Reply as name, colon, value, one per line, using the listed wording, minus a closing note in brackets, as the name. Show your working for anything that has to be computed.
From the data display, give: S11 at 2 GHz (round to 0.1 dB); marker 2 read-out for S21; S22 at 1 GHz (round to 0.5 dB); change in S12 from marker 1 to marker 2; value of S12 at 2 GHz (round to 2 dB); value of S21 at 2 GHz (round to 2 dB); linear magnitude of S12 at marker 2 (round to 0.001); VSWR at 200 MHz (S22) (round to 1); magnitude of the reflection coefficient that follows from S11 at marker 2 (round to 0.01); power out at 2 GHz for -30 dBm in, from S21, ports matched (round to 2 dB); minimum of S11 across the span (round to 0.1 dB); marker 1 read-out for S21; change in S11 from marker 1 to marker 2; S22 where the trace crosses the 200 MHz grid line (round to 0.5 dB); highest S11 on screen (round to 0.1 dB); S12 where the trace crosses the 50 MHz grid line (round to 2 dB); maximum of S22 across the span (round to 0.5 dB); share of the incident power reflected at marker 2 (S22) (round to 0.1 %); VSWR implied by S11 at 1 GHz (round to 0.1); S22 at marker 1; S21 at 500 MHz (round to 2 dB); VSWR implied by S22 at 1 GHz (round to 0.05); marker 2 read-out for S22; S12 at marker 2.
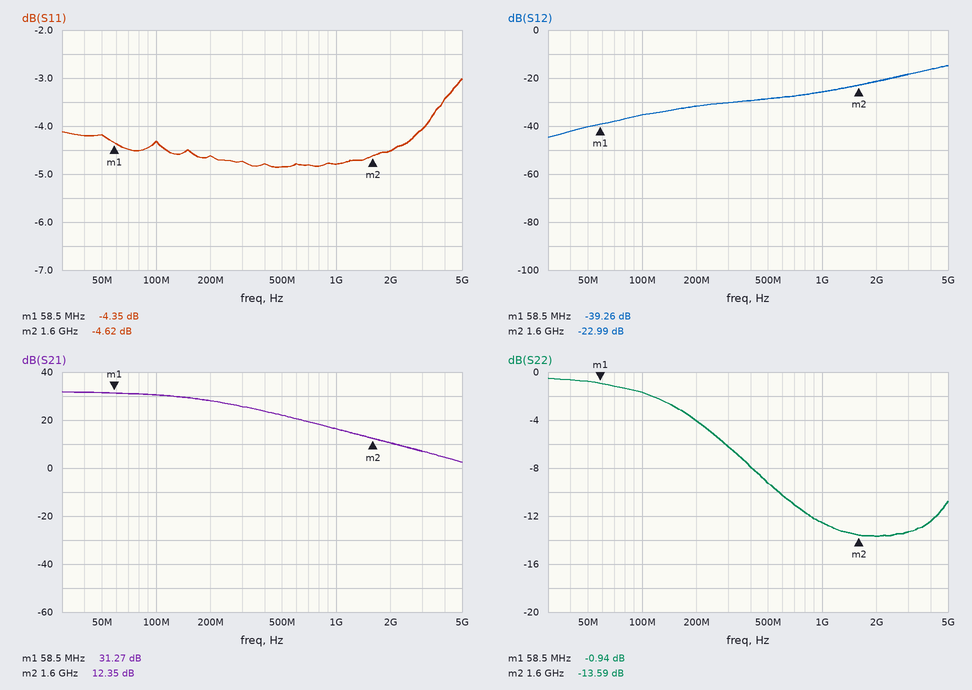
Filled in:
S11 at 2 GHz: -4.5 dB
marker 2 read-out for S21: 12.35 dB
S22 at 1 GHz: -12.5 dB
change in S12 from marker 1 to marker 2: -22.99 − (-39.26) = 16.27 dB
value of S12 at 2 GHz: -22 dB
value of S21 at 2 GHz: 10 dB
linear magnitude of S12 at marker 2: 10^(-22.99/20) ≈ 0.071
VSWR at 200 MHz (S22): |Γ| = 10^(-4/20) = 0.6310; VSWR = (1 + 0.6310)/(1 − 0.6310) ≈ 4
magnitude of the reflection coefficient that follows from S11 at marker 2: 10^(-4.62/20) ≈ 0.59
power out at 2 GHz for -30 dBm in, from S21, ports matched: -30 dBm + (10 dB) = -20 dBm
minimum of S11 across the span: -4.9 dB
marker 1 read-out for S21: 31.27 dB
change in S11 from marker 1 to marker 2: -4.62 − (-4.35) = -0.27 dB
S22 where the trace crosses the 200 MHz grid line: -4.0 dB
highest S11 on screen: -3.0 dB
S12 where the trace crosses the 50 MHz grid line: -40 dB
maximum of S22 across the span: -0.5 dB
share of the incident power reflected at marker 2 (S22): 10^(-13.59/10) ≈ 4.4 %
VSWR implied by S11 at 1 GHz: |Γ| = 10^(-4.8/20) = 0.5754; VSWR = (1 + 0.5754)/(1 − 0.5754) ≈ 3.7
S22 at marker 1: -0.94 dB
S21 at 500 MHz: 22 dB
VSWR implied by S22 at 1 GHz: |Γ| = 10^(-12.5/20) = 0.2371; VSWR = (1 + 0.2371)/(1 − 0.2371) ≈ 1.62, so 1.60 to the nearest 0.05
marker 2 read-out for S22: -13.59 dB
S12 at marker 2: -22.99 dB
